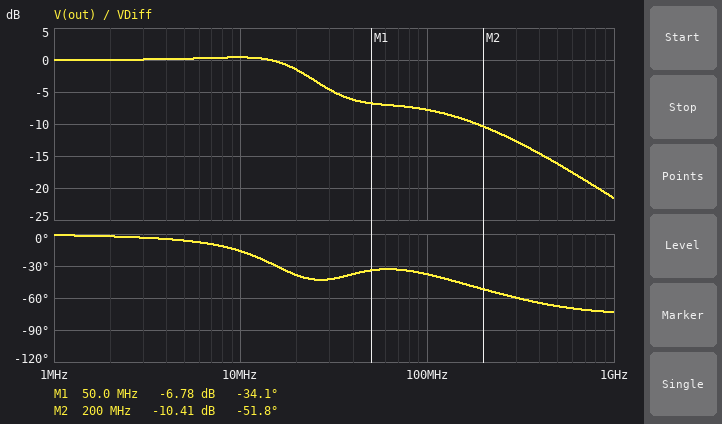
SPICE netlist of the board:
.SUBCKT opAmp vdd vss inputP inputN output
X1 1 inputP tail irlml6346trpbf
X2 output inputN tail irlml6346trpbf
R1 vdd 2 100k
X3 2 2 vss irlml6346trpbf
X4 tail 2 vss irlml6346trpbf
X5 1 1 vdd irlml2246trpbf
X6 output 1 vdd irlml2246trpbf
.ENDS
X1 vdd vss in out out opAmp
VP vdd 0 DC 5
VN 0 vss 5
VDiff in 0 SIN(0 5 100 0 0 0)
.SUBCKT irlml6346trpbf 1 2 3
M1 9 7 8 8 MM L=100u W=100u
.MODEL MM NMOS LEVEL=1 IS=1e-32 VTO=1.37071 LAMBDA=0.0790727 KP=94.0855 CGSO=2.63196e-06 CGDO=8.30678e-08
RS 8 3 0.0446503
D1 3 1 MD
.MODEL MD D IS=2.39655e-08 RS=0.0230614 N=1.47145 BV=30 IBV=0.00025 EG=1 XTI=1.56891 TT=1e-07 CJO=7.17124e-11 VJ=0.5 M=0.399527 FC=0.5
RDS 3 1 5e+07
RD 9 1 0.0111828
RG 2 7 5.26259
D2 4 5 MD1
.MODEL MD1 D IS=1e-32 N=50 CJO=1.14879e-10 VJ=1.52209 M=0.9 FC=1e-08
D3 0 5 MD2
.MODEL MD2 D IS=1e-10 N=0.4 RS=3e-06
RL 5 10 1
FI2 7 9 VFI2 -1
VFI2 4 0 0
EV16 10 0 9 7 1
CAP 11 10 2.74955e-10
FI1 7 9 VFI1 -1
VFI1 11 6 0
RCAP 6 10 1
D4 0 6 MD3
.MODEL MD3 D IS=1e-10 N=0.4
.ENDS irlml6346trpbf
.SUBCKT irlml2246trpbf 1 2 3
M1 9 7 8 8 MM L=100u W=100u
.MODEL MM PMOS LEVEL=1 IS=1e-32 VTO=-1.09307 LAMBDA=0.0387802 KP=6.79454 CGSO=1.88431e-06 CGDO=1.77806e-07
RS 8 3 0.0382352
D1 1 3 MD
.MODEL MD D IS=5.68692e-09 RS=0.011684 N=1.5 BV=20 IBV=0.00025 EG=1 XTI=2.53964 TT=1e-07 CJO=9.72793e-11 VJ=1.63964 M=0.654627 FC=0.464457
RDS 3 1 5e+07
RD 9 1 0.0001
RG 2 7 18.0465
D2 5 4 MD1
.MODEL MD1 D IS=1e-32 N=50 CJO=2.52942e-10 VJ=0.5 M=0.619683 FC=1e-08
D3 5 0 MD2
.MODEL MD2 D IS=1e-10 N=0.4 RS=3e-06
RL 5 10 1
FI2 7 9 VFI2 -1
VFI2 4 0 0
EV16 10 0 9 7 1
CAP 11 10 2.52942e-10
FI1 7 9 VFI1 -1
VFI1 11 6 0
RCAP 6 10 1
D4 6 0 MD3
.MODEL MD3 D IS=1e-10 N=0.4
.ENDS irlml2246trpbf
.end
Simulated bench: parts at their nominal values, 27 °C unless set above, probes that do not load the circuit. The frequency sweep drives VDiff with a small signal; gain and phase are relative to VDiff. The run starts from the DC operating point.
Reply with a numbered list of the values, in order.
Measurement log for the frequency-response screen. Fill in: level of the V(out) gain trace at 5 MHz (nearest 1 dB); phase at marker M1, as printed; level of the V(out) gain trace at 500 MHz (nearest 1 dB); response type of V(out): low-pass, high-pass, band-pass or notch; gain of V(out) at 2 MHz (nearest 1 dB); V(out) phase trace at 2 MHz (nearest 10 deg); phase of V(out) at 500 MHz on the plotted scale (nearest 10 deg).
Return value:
1. 0 dB
2. -34.1 deg
3. -16 dB
4. low-pass
5. 0 dB
6. 0 deg
7. -70 deg
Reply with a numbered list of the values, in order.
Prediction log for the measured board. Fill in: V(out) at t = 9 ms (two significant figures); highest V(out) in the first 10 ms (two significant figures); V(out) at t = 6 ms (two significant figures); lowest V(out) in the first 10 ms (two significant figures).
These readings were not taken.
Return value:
1. -2.9 V
2. 5.0 V
3. -2.9 V
4. -3.6 V
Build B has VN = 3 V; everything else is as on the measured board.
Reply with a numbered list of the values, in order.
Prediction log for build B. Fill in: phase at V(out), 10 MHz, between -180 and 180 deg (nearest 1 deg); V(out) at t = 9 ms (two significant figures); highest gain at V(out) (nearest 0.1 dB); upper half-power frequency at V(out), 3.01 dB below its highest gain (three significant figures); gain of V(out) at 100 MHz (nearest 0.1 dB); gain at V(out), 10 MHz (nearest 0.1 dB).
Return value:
1. -25 deg
2. -1.6 V
3. 0.7 dB
4. 17.6 MHz
5. -8.9 dB
6. 0.6 dB
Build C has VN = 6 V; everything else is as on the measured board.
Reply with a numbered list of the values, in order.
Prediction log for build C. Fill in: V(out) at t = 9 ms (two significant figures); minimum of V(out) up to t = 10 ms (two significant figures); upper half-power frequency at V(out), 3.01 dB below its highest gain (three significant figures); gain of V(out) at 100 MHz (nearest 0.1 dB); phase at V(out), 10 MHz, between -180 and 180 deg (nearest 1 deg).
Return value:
1. -2.9 V
2. -4.6 V
3. 25.4 MHz
4. -7.5 dB
5. -14 deg
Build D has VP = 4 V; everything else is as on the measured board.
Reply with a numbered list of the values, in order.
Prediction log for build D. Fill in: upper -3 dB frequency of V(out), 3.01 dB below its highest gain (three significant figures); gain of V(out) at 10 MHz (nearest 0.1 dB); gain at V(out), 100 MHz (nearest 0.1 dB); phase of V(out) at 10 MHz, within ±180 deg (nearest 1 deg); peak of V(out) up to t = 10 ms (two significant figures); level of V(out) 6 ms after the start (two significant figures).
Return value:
1. 20.4 MHz
2. 0.3 dB
3. -8.2 dB
4. -20 deg
5. 4.0 V
6. -2.9 V
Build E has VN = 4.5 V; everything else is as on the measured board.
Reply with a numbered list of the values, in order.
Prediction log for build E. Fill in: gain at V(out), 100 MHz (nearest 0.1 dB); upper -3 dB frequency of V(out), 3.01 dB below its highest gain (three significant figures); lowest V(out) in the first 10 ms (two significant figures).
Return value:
1. -8.0 dB
2. 21.8 MHz
3. -3.1 V
